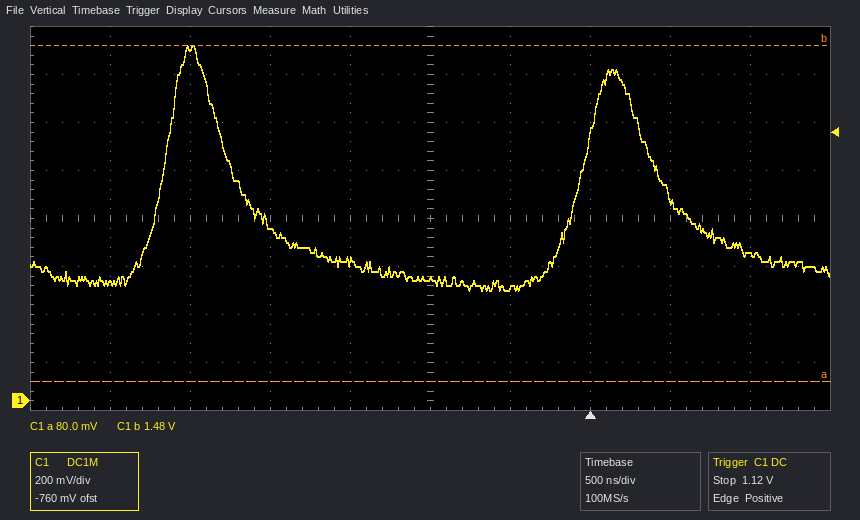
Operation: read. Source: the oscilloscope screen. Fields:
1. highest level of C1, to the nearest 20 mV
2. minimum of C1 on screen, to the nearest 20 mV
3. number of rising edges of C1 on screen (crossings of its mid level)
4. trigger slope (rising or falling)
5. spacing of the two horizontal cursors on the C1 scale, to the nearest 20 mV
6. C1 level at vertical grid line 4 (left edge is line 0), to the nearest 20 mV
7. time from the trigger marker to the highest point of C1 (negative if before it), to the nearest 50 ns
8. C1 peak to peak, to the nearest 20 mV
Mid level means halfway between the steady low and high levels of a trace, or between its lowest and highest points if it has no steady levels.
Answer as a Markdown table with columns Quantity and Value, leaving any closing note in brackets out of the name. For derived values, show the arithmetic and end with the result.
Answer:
| Quantity | Value |
|---|---|
| highest level of C1, to the nearest 20 mV | 1.48 V |
| minimum of C1 on screen, to the nearest 20 mV | 460 mV |
| number of rising edges of C1 on screen | 2 |
| trigger slope | rising |
| spacing of the two horizontal cursors on the C1 scale, to the nearest 20 mV | 1.40 V |
| C1 level at vertical grid line 4 (left edge is line 0), to the nearest 20 mV | 580 mV |
| time from the trigger marker to the highest point of C1 (negative if before it), to the nearest 50 ns | -2.50 µs |
| C1 peak to peak, to the nearest 20 mV | 1.48 V − (460 mV) = 1.02 V |
